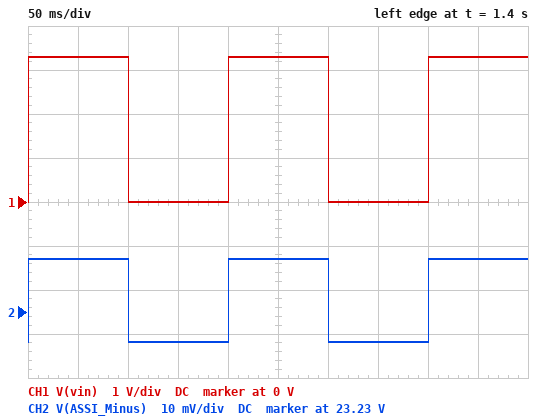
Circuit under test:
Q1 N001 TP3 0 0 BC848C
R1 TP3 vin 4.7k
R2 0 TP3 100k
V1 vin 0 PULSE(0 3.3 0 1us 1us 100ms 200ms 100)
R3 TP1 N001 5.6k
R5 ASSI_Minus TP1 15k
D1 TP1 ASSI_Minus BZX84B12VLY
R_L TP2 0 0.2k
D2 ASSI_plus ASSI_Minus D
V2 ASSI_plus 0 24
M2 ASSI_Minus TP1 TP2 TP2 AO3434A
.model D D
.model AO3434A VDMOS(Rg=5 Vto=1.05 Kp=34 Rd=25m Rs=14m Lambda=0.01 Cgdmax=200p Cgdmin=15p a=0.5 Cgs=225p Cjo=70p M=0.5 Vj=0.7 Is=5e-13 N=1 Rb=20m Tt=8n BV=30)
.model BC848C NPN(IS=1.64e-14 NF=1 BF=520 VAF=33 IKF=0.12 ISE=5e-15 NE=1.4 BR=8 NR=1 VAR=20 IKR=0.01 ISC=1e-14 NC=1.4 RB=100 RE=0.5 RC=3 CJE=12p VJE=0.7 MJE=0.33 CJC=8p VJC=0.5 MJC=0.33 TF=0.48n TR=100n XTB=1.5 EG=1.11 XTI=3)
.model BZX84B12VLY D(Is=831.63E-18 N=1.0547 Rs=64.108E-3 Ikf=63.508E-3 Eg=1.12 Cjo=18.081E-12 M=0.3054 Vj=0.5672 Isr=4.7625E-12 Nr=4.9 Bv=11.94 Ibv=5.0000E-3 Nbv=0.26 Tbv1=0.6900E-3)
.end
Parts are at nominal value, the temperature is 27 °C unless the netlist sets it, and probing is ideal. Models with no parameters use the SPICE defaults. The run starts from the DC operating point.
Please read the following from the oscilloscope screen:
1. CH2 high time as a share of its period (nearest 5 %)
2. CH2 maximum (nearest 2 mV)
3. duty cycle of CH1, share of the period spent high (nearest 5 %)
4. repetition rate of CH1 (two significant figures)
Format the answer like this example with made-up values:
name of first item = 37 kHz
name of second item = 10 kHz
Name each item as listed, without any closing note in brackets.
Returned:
CH2 high time as a share of its period = 50 %
CH2 maximum = 23.242 V
duty cycle of CH1, share of the period spent high = 50 %
repetition rate of CH1 = 5.0 Hz
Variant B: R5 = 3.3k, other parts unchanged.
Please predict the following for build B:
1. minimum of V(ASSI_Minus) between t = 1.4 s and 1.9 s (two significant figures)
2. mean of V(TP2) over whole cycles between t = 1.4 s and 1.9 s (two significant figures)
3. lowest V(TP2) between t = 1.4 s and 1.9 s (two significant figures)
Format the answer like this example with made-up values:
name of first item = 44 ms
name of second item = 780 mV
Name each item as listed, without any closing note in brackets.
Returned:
minimum of V(ASSI_Minus) between t = 1.4 s and 1.9 s = 23 V
mean of V(TP2) over whole cycles between t = 1.4 s and 1.9 s = 18 V
lowest V(TP2) between t = 1.4 s and 1.9 s = 14 V
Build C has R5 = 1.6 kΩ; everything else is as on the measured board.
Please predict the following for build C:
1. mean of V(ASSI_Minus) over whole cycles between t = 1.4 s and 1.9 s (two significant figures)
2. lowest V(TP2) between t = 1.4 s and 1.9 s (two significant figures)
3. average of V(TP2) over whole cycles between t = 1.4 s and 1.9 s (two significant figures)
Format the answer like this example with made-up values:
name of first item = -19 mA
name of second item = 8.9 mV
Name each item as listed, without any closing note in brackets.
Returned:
mean of V(ASSI_Minus) over whole cycles between t = 1.4 s and 1.9 s = 23 V
lowest V(TP2) between t = 1.4 s and 1.9 s = 17 V
average of V(TP2) over whole cycles between t = 1.4 s and 1.9 s = 20 V
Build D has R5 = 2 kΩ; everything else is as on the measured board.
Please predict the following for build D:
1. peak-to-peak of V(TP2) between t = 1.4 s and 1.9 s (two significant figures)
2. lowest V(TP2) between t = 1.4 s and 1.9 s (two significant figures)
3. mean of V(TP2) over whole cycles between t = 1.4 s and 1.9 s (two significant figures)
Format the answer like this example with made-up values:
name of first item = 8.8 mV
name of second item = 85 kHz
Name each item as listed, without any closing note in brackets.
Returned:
peak-to-peak of V(TP2) between t = 1.4 s and 1.9 s = 6.1 V
lowest V(TP2) between t = 1.4 s and 1.9 s = 16 V
mean of V(TP2) over whole cycles between t = 1.4 s and 1.9 s = 19 V
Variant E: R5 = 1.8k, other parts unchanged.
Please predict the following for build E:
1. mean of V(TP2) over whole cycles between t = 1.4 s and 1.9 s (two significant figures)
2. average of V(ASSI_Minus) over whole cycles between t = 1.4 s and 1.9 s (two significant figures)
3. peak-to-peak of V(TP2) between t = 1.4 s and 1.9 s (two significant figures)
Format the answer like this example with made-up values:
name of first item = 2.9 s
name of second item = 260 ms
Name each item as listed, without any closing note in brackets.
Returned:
mean of V(TP2) over whole cycles between t = 1.4 s and 1.9 s = 19 V
average of V(ASSI_Minus) over whole cycles between t = 1.4 s and 1.9 s = 23 V
peak-to-peak of V(TP2) between t = 1.4 s and 1.9 s = 5.6 V
